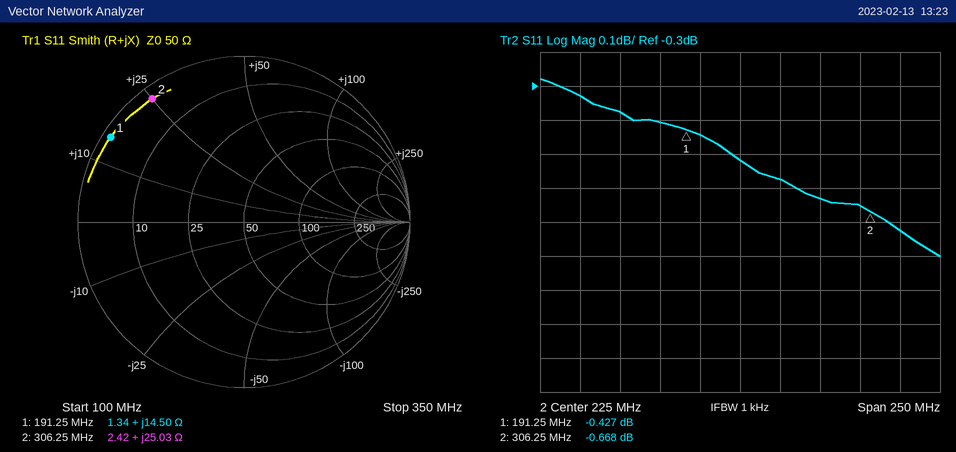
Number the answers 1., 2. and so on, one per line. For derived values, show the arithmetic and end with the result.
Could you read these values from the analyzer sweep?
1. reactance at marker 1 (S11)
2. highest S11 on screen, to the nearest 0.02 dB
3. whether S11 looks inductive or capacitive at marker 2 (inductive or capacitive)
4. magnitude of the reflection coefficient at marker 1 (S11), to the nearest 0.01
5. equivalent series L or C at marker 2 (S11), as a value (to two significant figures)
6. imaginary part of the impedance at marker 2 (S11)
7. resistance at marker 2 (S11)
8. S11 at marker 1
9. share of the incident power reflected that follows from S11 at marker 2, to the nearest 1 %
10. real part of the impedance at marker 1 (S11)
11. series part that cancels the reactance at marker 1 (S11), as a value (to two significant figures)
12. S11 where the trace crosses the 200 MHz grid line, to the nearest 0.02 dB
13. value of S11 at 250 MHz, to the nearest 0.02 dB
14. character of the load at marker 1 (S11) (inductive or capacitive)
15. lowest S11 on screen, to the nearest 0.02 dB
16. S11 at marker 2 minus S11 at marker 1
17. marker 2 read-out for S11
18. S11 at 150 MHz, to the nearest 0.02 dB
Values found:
1. +14.50 Ω
2. -0.28 dB
3. inductive
4. 0.95
5. L = 25.03 Ω/(2π × 306.25 MHz) ≈ 13 nH
6. +25.03 Ω
7. 2.42 Ω
8. -0.427 dB
9. 10^(-0.668/10) ≈ 86 %
10. 1.34 Ω
11. C = 1/(2π × 191.25 MHz × 14.5 Ω) ≈ 57 pF
12. -0.44 dB
13. -0.58 dB
14. inductive
15. -0.80 dB
16. -0.668 − (-0.427) = -0.241 dB
17. -0.668 dB
18. -0.38 dB
